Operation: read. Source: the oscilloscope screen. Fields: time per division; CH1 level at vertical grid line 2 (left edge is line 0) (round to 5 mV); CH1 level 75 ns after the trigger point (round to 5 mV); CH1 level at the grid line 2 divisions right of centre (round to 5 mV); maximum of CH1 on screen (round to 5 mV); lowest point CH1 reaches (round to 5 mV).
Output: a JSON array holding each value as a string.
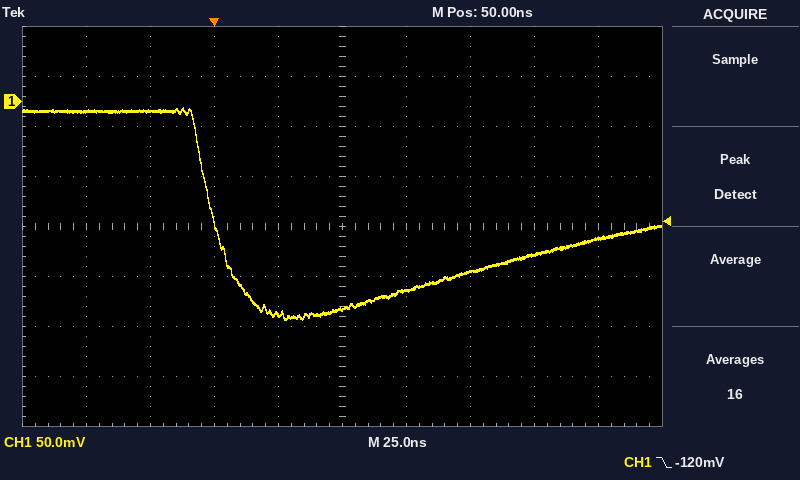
["25 ns", "-10 mV", "-190 mV", "-170 mV", "-5 mV", "-220 mV"]
